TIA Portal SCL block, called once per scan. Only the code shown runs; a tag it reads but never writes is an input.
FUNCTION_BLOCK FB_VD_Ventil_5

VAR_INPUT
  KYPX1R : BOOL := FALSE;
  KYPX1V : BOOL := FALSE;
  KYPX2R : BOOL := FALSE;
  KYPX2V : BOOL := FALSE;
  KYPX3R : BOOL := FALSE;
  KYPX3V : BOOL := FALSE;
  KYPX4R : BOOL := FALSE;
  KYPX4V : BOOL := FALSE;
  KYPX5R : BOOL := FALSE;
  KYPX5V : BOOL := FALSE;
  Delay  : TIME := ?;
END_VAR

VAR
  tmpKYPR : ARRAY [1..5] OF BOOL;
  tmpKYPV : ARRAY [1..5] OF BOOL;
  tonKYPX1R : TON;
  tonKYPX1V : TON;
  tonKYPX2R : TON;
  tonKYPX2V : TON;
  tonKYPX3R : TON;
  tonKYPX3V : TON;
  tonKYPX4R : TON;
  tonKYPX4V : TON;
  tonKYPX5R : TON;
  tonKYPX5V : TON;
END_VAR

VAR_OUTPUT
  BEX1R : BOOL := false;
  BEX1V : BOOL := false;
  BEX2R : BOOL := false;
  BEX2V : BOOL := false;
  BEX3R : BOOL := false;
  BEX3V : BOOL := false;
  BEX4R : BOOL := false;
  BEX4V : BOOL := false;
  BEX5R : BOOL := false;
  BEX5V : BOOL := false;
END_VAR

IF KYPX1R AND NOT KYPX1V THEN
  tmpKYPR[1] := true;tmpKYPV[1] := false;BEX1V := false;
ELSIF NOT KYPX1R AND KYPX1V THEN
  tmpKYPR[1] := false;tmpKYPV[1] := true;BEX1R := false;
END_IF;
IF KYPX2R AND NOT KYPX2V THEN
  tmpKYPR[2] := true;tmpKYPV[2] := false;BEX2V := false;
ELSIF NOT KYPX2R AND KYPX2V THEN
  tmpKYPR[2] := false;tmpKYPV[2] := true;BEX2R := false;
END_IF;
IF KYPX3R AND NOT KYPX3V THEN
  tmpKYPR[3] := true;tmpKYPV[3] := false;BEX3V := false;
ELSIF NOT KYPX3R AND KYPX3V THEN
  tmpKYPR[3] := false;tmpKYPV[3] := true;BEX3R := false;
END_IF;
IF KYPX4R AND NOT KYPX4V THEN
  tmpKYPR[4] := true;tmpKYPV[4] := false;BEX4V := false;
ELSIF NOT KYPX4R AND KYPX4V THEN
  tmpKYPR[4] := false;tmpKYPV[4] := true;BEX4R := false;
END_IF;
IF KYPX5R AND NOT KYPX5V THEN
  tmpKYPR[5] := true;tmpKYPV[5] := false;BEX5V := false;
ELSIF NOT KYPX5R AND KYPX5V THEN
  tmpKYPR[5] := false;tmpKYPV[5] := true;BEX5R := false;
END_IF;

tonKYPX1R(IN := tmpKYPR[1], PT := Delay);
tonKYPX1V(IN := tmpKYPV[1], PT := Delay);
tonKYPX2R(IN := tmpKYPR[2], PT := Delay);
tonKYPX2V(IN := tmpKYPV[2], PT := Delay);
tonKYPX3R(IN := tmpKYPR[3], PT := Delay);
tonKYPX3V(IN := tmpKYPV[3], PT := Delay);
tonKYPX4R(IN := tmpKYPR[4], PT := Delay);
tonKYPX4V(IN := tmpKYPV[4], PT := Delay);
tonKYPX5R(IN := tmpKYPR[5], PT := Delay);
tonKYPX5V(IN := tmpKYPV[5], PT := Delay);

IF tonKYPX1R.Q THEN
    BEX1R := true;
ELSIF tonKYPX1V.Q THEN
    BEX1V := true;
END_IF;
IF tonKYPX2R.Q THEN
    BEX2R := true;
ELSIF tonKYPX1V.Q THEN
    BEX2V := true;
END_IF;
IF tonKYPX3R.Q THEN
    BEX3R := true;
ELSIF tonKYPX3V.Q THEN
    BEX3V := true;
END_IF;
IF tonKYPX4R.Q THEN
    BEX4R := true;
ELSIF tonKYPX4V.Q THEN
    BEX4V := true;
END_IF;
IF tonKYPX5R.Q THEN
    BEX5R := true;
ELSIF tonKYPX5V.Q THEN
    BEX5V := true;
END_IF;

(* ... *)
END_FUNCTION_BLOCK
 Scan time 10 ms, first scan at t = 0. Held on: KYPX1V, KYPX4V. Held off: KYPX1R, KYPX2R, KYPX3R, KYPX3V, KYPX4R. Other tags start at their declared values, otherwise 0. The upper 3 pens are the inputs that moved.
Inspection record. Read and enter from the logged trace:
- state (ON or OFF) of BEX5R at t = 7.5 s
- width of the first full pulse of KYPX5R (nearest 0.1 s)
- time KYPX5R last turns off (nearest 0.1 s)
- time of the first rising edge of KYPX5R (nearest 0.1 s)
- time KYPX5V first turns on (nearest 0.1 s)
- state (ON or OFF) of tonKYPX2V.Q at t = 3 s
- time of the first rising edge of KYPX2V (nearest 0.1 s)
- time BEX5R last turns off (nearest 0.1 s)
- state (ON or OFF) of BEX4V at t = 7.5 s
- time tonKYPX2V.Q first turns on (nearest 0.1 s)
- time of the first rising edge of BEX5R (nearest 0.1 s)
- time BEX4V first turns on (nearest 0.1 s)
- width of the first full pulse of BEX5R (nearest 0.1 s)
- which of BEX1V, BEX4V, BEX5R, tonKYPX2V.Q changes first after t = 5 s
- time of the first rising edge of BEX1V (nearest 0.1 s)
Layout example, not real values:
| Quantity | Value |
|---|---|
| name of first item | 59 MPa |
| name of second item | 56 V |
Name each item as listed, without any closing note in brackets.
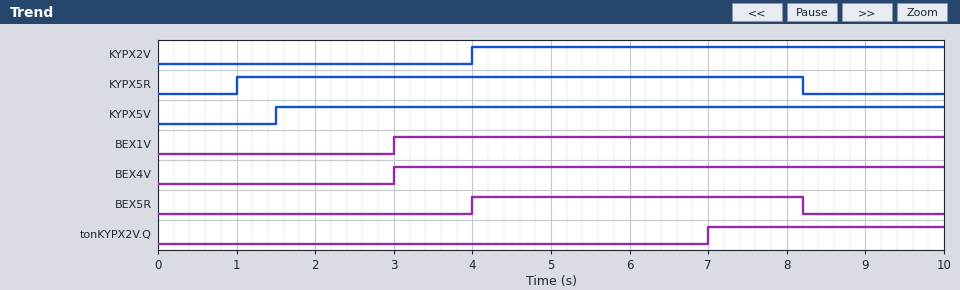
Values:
| Quantity | Value |
|---|---|
| state (ON or OFF) of BEX5R at t = 7.5 s | ON |
| width of the first full pulse of KYPX5R | 7.2 s |
| time KYPX5R last turns off | 8.2 s |
| time of the first rising edge of KYPX5R | 1.0 s |
| time KYPX5V first turns on | 1.5 s |
| state (ON or OFF) of tonKYPX2V.Q at t = 3 s | OFF |
| time of the first rising edge of KYPX2V | 4.0 s |
| time BEX5R last turns off | 8.2 s |
| state (ON or OFF) of BEX4V at t = 7.5 s | ON |
| time tonKYPX2V.Q first turns on | 7.0 s |
| time of the first rising edge of BEX5R | 4.0 s |
| time BEX4V first turns on | 3.0 s |
| width of the first full pulse of BEX5R | 4.2 s |
| which of BEX1V, BEX4V, BEX5R, tonKYPX2V.Q changes first after t = 5 s | tonKYPX2V.Q |
| time of the first rising edge of BEX1V | 3.0 s |
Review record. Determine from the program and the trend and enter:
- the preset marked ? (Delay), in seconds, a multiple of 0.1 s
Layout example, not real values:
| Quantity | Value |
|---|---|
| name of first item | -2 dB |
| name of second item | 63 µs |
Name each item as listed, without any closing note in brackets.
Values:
| Quantity | Value |
|---|---|
| the preset marked ? (Delay), in seconds, a multiple of 0.1 s | 3.0 s |
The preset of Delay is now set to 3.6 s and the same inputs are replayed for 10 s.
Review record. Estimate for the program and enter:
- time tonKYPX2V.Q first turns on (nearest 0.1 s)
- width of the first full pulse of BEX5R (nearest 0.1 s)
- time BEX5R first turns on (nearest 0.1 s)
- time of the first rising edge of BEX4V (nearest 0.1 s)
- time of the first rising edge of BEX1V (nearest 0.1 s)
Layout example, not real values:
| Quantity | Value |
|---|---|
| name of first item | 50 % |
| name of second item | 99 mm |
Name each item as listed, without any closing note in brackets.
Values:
| Quantity | Value |
|---|---|
| time tonKYPX2V.Q first turns on | 7.6 s |
| width of the first full pulse of BEX5R | 3.6 s |
| time BEX5R first turns on | 4.6 s |
| time of the first rising edge of BEX4V | 3.6 s |
| time of the first rising edge of BEX1V | 3.6 s |
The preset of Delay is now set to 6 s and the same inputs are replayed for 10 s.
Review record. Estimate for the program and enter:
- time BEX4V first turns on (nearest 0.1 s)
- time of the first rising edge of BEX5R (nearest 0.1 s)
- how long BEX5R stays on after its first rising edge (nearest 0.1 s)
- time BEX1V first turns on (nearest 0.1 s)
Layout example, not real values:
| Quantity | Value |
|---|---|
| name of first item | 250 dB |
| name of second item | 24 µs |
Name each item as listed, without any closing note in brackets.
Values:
| Quantity | Value |
|---|---|
| time BEX4V first turns on | 6.0 s |
| time of the first rising edge of BEX5R | 7.0 s |
| how long BEX5R stays on after its first rising edge | 1.2 s |
| time BEX1V first turns on | 6.0 s |
